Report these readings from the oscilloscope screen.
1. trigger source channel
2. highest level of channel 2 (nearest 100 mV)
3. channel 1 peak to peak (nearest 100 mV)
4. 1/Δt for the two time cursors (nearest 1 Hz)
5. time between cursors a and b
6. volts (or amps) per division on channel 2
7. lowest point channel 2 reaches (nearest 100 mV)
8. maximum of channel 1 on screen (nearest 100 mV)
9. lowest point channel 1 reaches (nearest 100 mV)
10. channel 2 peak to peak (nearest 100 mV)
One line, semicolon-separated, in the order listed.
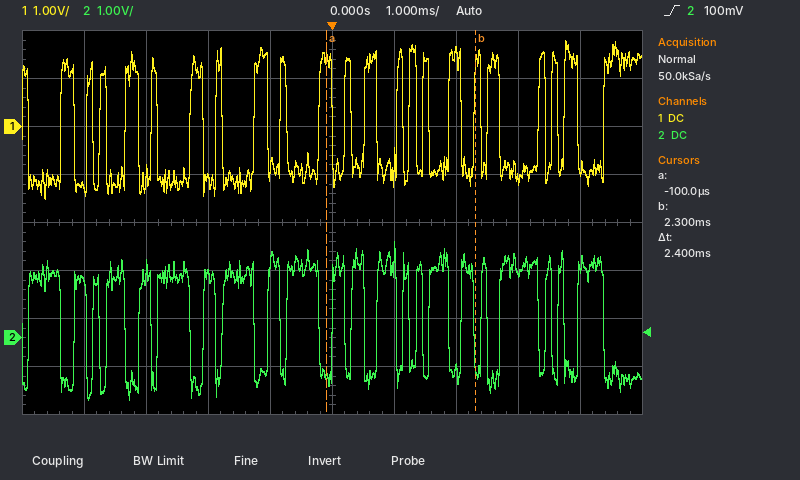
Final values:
channel 2; 2.0 V; 3.3 V; 417 Hz; 2.4 ms; 1 V; -1.3 V; 1.8 V; -1.5 V; 3.3 V
